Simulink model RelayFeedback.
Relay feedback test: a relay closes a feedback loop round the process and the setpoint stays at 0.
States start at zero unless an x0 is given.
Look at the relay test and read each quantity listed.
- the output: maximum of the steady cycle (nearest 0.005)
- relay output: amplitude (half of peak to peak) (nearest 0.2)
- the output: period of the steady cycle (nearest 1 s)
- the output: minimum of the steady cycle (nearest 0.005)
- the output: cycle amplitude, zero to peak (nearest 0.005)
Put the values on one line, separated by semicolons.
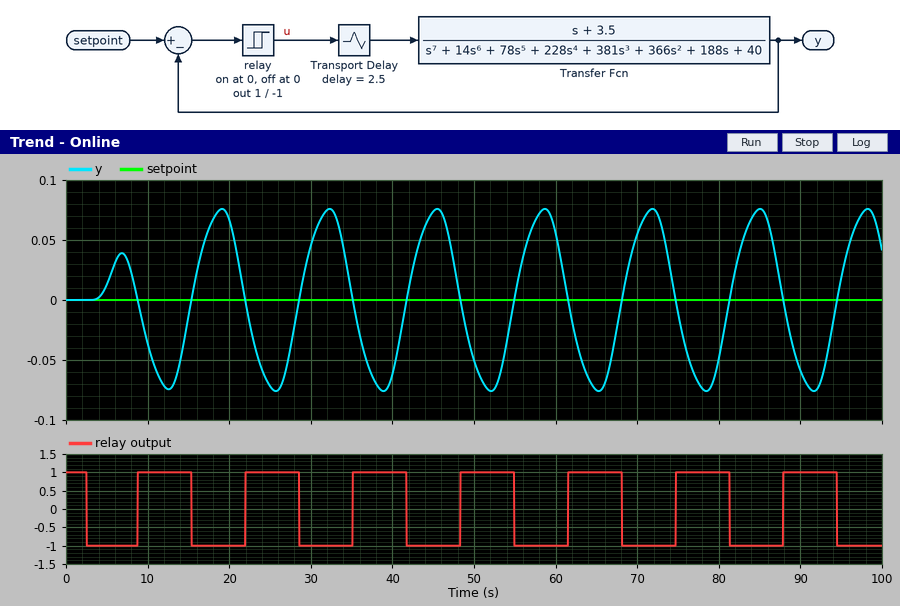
0.075; 1.0; 13 s; -0.075; 0.075
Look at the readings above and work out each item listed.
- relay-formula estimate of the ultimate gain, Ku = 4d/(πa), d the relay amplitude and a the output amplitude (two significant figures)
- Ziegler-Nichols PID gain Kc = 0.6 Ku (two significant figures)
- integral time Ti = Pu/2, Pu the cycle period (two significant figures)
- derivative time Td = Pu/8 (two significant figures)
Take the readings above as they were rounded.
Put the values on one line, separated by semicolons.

17; 10; 6.5 s; 1.6 s
